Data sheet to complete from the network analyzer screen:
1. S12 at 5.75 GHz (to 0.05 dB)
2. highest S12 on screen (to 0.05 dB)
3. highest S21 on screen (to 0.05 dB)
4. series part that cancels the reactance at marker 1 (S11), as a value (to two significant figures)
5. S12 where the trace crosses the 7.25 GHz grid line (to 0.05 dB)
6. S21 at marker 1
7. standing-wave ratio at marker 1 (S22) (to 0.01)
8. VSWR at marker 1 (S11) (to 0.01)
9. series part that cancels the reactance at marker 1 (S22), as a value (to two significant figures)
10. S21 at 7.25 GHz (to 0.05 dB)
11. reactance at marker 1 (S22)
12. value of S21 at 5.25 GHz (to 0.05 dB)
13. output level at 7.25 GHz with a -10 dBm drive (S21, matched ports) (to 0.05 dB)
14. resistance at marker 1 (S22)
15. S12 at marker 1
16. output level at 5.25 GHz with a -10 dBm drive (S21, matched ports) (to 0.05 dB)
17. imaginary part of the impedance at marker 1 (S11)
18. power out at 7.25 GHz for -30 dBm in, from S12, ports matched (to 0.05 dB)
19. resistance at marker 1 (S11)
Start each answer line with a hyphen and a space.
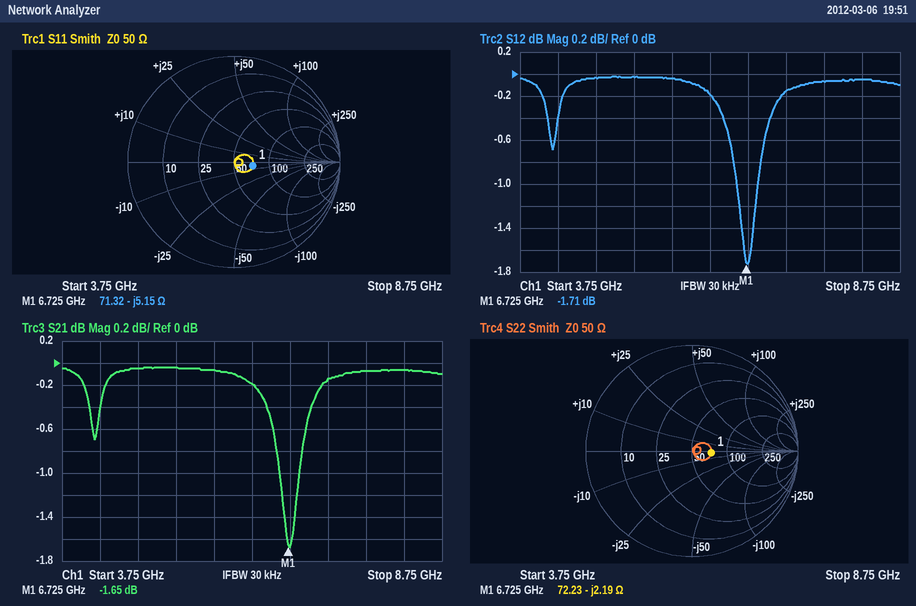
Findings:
- -0.05 dB
- 0.00 dB
- -0.05 dB
- 120 pH
- -0.15 dB
- -1.65 dB
- 1.45
- 1.44
- 52 pH
- -0.15 dB
- -2.19 Ω
- -0.05 dB
- -10.15 dBm
- 72.23 Ω
- -1.71 dB
- -10.05 dBm
- -5.15 Ω
- -30.15 dBm
- 71.32 Ω
